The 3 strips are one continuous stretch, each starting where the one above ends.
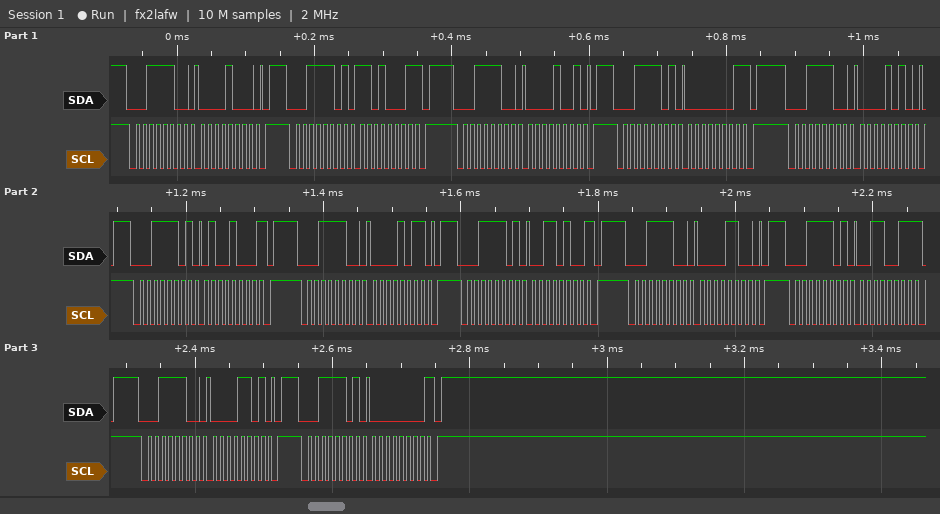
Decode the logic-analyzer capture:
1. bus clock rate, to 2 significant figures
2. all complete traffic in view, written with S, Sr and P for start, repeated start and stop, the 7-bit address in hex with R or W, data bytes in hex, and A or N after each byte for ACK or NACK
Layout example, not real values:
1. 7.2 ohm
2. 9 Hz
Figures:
1. 100 kHz
2. S 1EW A 08 A P S 1ER A D1 N P S 1EW A 09 A P S 1ER A 01 N P S 1EW A 0A A P S 1ER A 48 N P S 1EW A 0B A P S 1ER A 34 N P S 1EW A 0C A P S 1ER A 33 N P S 1EW A 0D A P S 1ER A 00 N P
